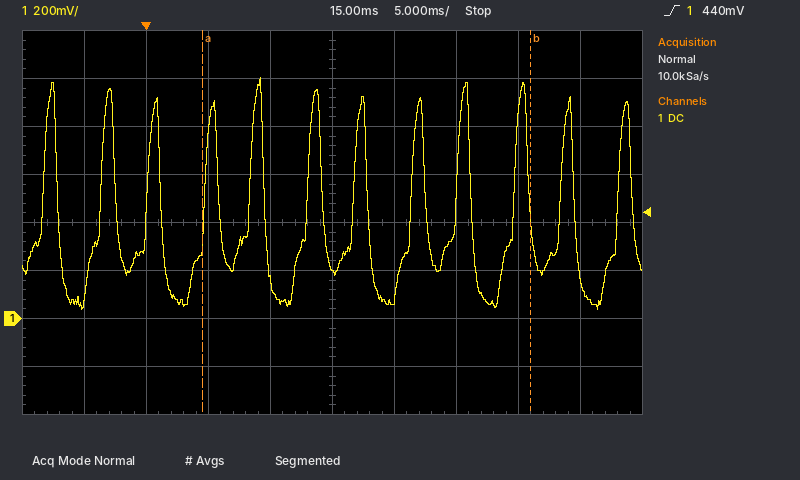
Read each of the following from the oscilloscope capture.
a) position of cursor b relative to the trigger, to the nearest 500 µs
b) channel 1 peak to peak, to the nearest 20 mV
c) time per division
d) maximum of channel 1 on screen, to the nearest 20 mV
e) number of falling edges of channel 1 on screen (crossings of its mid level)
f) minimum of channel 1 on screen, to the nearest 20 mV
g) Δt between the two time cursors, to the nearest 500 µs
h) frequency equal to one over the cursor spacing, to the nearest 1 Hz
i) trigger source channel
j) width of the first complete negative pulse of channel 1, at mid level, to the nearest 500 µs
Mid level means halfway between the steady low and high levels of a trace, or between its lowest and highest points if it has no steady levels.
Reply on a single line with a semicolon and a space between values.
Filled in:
+31.0 ms; 960 mV; 5 ms; 1.00 V; 12; 40 mV; 26.5 ms; 38 Hz; channel 1; 3.5 ms
